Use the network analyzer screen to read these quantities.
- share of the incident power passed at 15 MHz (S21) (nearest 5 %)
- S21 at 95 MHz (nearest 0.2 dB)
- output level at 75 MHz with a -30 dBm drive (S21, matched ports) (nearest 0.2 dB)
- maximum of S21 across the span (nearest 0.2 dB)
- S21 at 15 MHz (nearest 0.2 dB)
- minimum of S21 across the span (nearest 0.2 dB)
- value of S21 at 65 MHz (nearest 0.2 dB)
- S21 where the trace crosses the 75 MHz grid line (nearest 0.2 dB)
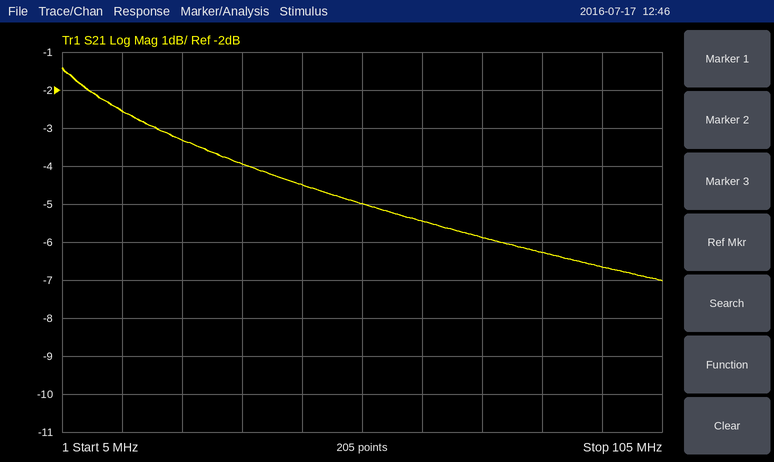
55 %
-6.6 dB
-35.8 dBm
-1.4 dB
-2.6 dB
-7.0 dB
-5.4 dB
-5.8 dB
